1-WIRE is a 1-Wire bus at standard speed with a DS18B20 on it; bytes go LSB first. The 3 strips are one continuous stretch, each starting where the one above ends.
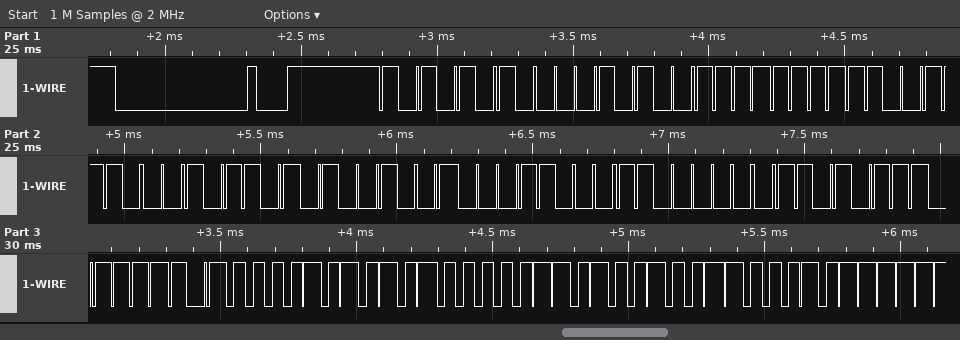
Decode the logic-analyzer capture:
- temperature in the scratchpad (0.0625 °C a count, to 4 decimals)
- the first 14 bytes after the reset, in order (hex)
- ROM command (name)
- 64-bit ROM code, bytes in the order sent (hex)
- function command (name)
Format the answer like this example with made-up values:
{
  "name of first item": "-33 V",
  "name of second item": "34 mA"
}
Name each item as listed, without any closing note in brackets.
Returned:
{
  "temperature in the scratchpad": "85.0000 °C",
  "the first 14 bytes after the reset, in order": "55 28 FF 73 B4 92 18 03 EB BE 50 05 4B 46",
  "ROM command": "Match ROM",
  "64-bit ROM code, bytes in the order sent": "28 FF 73 B4 92 18 03 EB",
  "function command": "Read Scratchpad"
}
